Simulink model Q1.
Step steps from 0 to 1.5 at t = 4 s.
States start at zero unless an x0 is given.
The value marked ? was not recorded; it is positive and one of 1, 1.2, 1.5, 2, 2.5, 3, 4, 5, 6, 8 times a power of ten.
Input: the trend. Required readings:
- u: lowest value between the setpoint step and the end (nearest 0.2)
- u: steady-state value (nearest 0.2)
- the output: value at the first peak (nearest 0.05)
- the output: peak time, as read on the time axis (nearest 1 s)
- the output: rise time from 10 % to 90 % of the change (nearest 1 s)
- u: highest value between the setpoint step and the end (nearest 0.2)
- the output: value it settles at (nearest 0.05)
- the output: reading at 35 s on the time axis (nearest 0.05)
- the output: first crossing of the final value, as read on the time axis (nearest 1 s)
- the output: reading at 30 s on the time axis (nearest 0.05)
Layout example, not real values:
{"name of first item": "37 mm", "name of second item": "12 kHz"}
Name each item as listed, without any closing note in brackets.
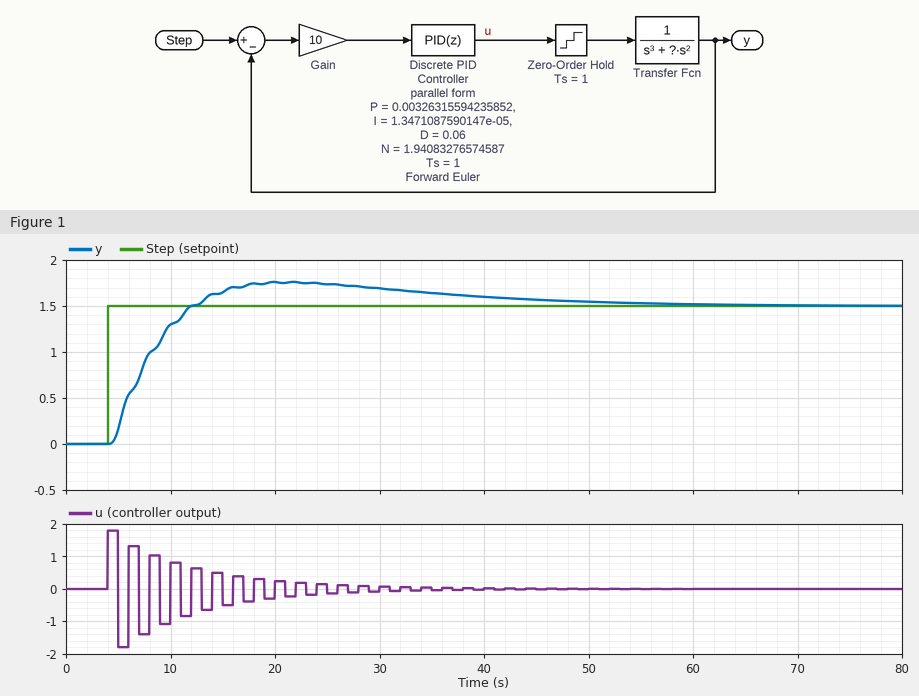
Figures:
{"u: lowest value between the setpoint step and the end": "-1.8", "u: steady-state value": "0.0", "the output: value at the first peak": "1.75", "the output: peak time, as read on the time axis": "22 s", "the output: rise time from 10 % to 90 % of the change": "6 s", "u: highest value between the setpoint step and the end": "1.8", "the output: value it settles at": "1.50", "the output: reading at 35 s on the time axis": "1.65", "the output: first crossing of the final value, as read on the time axis": "12 s", "the output: reading at 30 s on the time axis": "1.70"}
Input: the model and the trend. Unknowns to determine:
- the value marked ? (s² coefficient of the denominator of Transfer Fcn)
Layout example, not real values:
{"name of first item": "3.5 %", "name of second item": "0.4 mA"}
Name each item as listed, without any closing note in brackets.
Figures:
{"the value marked ?": "3"}
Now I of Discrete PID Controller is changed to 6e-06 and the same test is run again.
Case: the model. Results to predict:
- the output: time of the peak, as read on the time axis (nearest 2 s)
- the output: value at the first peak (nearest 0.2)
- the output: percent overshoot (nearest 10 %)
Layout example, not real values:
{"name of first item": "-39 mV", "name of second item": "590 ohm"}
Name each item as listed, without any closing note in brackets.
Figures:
{"the output: time of the peak, as read on the time axis": "20 s", "the output: value at the first peak": "1.8", "the output: percent overshoot": "20 %"}
